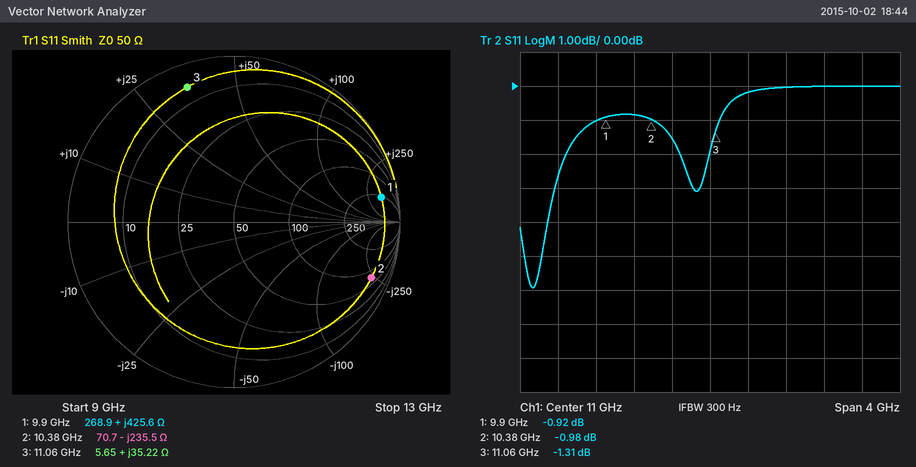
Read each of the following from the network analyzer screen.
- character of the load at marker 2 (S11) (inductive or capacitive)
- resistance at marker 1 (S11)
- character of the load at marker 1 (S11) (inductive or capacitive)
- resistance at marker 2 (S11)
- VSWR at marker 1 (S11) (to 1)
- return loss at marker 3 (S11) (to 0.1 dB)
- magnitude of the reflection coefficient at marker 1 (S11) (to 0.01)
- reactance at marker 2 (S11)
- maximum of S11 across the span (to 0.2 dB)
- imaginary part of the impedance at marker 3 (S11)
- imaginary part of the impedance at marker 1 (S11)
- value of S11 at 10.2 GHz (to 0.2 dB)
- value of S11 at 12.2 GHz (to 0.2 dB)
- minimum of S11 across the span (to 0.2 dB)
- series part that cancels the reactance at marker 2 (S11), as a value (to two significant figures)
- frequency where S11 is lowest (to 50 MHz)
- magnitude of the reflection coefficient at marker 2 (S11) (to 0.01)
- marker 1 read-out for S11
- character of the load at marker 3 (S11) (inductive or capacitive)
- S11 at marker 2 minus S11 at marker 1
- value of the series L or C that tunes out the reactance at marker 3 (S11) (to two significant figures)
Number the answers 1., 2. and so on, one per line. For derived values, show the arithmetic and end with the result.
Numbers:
1. capacitive
2. 268.9 Ω
3. inductive
4. 70.7 Ω
5. 19
6. 1.3 dB
7. 10^(-0.92/20) ≈ 0.90
8. -235.5 Ω
9. 0.0 dB
10. +35.22 Ω
11. +425.6 Ω
12. -0.8 dB
13. 0.0 dB
14. -6.0 dB
15. L = 235.5 Ω/(2π × 10.38 GHz) ≈ 3.6 nH
16. 9.15 GHz
17. 0.89
18. -0.92 dB
19. inductive
20. -0.98 − (-0.92) = -0.06 dB
21. C = 1/(2π × 11.06 GHz × 35.22 Ω) ≈ 409 fF, so 410 fF to two significant figures
